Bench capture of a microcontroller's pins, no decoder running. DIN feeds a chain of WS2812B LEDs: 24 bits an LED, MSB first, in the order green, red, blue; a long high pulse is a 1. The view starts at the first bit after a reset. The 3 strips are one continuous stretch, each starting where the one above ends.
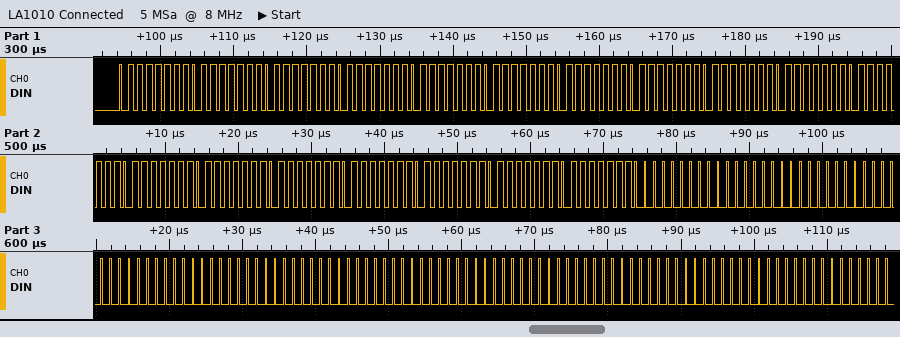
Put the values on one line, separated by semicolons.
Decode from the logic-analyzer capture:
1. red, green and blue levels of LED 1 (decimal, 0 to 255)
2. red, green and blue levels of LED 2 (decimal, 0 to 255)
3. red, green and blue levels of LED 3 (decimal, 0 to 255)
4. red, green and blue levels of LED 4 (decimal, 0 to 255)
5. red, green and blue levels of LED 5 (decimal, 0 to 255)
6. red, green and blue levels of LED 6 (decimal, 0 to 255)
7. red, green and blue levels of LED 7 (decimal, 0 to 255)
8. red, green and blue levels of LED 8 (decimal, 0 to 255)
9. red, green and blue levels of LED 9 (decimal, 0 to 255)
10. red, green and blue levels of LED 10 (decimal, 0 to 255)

127, 127, 127; 127, 127, 127; 127, 127, 127; 127, 127, 127; 127, 127, 127; 127, 127, 127; 0, 0, 0; 0, 0, 0; 0, 0, 0; 0, 0, 0
